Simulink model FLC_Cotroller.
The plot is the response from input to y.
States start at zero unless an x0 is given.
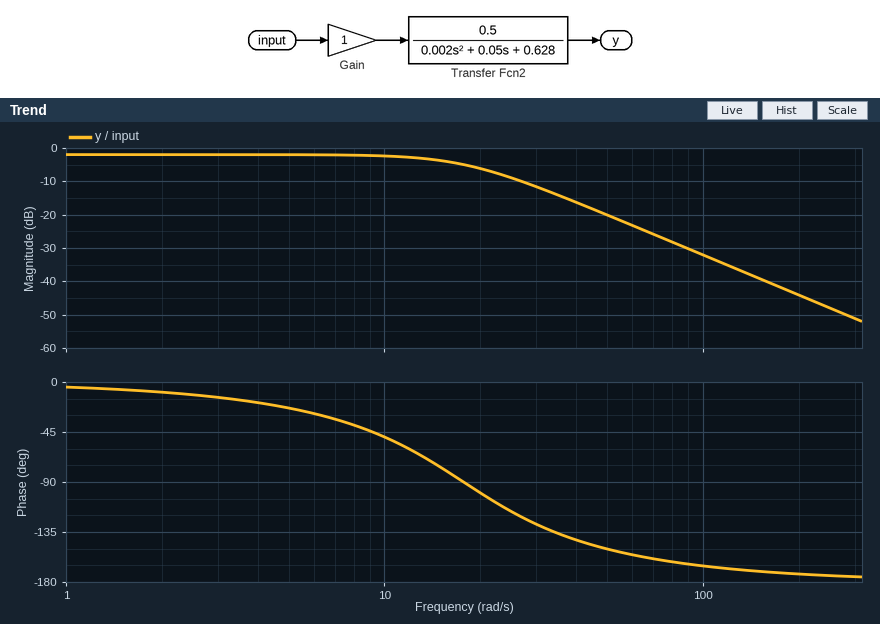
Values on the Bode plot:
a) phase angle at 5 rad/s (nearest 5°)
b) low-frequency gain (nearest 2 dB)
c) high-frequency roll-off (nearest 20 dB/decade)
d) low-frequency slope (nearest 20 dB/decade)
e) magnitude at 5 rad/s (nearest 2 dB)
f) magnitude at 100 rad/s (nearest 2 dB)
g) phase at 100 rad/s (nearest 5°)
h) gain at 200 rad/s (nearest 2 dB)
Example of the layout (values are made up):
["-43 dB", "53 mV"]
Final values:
["-25°", "-2 dB", "-40 dB/decade", "0 dB/decade", "-2 dB", "-32 dB", "-165°", "-44 dB"]
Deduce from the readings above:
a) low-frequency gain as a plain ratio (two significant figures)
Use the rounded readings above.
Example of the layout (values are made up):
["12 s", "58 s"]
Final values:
["0.79"]
